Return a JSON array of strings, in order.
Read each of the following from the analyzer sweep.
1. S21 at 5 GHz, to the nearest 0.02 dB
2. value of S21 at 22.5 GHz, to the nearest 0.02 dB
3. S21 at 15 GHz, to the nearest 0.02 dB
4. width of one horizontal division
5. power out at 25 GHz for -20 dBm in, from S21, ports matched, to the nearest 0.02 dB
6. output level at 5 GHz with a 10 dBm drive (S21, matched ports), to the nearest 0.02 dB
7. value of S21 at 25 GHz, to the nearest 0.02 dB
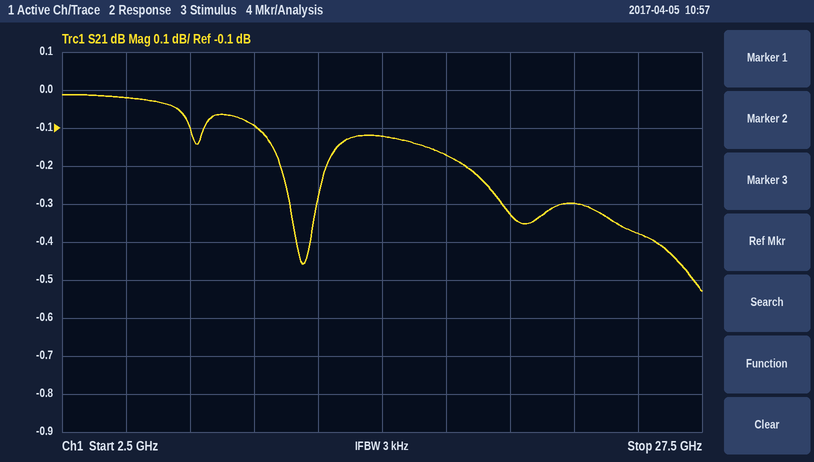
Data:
["-0.02 dB", "-0.30 dB", "-0.12 dB", "2.5 GHz", "-20.38 dBm", "9.98 dBm", "-0.38 dB"]
